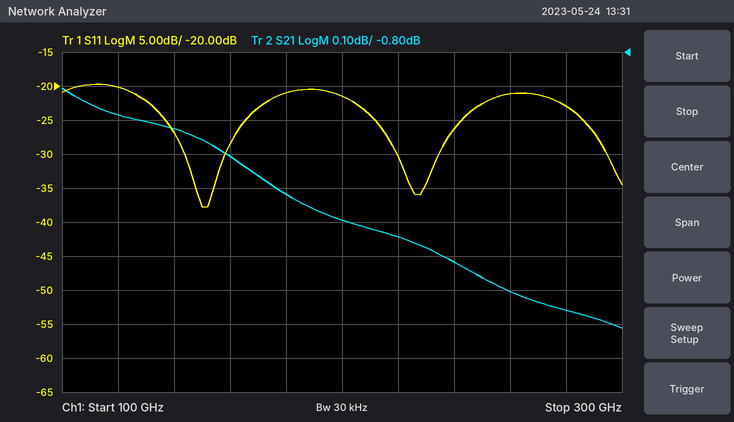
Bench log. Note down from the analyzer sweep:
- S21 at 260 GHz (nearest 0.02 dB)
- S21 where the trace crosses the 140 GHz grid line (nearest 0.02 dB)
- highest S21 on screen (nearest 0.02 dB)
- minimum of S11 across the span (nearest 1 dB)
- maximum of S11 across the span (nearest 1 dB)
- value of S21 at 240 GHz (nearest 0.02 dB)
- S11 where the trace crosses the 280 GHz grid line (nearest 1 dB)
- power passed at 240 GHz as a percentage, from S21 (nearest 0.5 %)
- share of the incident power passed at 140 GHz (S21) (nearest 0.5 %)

-1.50 dB
-1.02 dB
-0.90 dB
-38 dB
-20 dB
-1.42 dB
-23 dB
72.0 %
79.0 %
